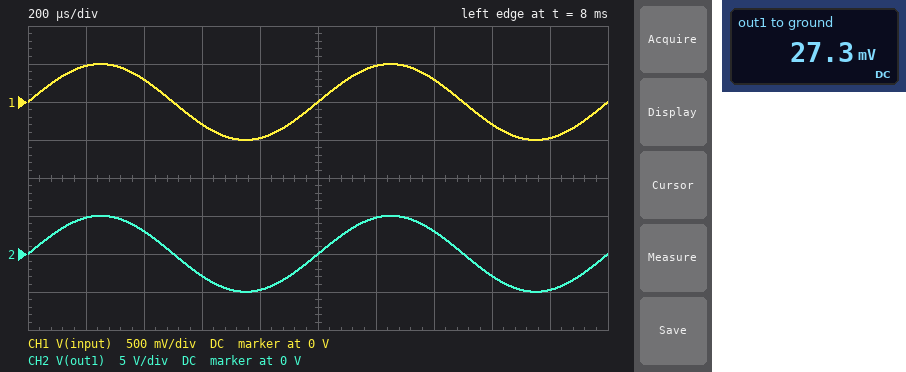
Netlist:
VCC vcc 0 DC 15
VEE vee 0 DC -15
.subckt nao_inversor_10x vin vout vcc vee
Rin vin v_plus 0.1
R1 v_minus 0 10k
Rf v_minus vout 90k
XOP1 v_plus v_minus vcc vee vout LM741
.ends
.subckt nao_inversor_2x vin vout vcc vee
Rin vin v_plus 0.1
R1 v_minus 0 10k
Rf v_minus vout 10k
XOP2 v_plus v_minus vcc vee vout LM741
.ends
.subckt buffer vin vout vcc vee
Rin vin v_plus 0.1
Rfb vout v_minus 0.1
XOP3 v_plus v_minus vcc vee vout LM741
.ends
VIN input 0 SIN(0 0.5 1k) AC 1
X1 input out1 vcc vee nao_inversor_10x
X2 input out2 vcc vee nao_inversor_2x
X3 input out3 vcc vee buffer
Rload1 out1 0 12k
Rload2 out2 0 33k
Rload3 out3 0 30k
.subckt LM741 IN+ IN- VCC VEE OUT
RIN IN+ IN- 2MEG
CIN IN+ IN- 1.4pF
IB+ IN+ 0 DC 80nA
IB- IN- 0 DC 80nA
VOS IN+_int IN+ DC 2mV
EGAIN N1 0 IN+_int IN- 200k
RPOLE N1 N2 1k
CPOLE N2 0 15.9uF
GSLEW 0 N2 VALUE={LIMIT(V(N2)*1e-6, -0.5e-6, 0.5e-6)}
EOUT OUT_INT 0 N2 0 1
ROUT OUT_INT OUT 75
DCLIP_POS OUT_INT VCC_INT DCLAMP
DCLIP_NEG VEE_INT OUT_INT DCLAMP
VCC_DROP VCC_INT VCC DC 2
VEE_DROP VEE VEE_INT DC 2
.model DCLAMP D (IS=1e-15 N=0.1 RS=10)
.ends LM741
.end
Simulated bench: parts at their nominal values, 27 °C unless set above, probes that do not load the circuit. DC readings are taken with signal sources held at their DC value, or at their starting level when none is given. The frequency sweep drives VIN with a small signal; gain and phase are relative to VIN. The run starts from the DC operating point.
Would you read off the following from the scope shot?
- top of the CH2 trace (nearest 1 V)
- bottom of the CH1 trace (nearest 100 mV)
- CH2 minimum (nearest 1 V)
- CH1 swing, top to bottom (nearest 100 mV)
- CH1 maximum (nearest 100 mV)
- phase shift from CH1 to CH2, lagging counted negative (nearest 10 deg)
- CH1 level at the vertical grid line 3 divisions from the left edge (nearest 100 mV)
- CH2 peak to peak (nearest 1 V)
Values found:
5 V
-500 mV
-5 V
1.0 V
500 mV
0 deg
-300 mV
10 V
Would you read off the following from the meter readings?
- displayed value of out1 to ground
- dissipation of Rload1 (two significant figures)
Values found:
27.3 mV
62 nW
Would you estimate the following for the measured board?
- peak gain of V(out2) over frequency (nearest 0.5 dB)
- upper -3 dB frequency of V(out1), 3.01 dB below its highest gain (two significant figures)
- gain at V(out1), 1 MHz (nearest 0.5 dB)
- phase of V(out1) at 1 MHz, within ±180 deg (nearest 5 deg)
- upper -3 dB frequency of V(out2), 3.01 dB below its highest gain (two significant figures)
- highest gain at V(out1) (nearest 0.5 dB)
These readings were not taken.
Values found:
6.0 dB
200 kHz
6.0 dB
-85 deg
1.0 MHz
20.0 dB
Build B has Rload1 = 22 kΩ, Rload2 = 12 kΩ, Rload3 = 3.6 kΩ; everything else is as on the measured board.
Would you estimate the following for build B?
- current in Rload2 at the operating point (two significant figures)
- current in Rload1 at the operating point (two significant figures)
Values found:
400 nA
1.2 µA
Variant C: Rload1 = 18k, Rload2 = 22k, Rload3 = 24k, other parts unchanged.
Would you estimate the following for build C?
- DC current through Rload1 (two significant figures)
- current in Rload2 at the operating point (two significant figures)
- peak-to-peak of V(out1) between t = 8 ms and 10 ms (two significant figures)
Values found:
1.5 µA
220 nA
10 V
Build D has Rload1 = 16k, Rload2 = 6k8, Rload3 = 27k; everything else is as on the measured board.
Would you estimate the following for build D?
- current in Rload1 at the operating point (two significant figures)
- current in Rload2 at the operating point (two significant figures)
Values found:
1.7 µA
710 nA
